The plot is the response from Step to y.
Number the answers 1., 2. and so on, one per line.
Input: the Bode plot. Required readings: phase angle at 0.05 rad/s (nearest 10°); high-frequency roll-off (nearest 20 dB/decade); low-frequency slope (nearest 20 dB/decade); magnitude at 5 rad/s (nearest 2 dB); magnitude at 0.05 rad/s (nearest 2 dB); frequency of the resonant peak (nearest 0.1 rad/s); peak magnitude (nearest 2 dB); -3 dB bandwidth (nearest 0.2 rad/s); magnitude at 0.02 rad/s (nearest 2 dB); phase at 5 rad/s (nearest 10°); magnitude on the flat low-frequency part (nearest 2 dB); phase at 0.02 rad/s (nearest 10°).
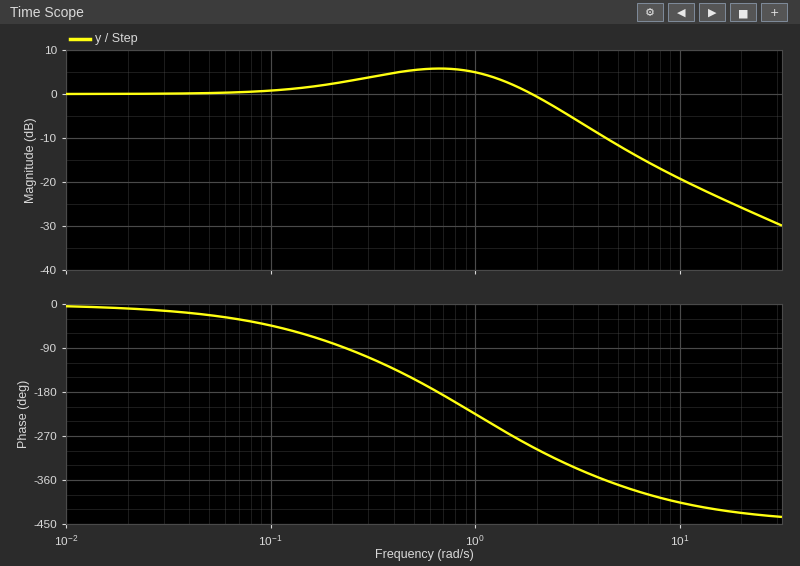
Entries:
1. -20°
2. -20 dB/decade
3. 0 dB/decade
4. -12 dB
5. 0 dB
6. 0.7 rad/s
7. 6 dB
8. 2.4 rad/s
9. 0 dB
10. -370°
11. 0 dB
12. -10°
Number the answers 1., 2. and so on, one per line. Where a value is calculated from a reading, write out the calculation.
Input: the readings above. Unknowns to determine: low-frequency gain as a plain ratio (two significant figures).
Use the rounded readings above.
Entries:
1. 10^(0 / 20) = 1.0
